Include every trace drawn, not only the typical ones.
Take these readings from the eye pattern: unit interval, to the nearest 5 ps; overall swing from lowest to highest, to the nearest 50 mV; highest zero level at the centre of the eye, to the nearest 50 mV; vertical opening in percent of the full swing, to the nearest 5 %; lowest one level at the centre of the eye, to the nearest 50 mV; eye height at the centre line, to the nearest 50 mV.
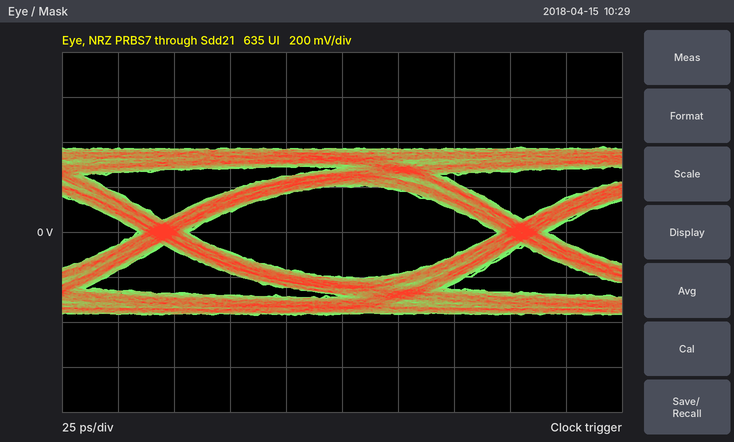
160 ps
750 mV
-200 mV
55 %
200 mV
400 mV
